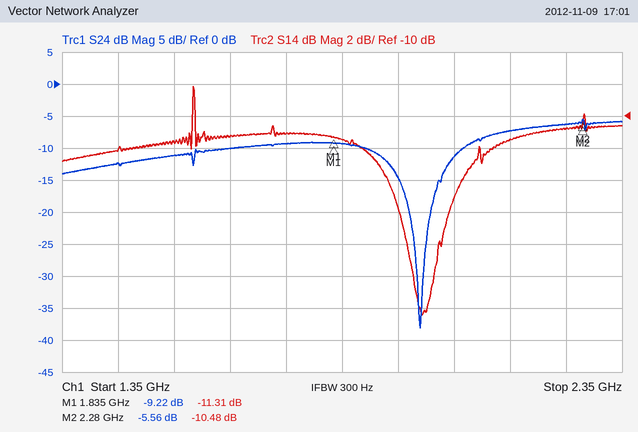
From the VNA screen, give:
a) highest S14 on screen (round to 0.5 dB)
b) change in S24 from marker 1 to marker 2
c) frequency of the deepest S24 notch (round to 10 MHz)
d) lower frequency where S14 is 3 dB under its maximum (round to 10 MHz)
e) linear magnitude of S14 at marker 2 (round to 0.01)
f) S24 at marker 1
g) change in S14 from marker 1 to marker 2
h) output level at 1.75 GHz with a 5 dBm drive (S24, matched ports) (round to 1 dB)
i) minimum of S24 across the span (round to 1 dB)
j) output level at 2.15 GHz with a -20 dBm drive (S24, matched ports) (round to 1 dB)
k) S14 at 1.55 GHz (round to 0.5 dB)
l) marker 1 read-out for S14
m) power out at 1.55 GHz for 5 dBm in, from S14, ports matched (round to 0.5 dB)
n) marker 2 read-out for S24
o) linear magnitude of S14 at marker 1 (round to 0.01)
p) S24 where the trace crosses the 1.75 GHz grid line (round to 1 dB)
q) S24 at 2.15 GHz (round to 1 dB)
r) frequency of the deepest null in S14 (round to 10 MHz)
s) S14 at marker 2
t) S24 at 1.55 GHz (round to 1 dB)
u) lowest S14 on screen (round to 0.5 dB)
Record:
-8.0 dB
3.66 dB
1.99 GHz
1.58 GHz
0.30
-9.22 dB
0.83 dB
-4 dBm
-38 dB
-27 dBm
-11.5 dB
-11.31 dB
-6.5 dBm
-5.56 dB
0.27
-9 dB
-7 dB
1.99 GHz
-10.48 dB
-11 dB
-22.5 dB
